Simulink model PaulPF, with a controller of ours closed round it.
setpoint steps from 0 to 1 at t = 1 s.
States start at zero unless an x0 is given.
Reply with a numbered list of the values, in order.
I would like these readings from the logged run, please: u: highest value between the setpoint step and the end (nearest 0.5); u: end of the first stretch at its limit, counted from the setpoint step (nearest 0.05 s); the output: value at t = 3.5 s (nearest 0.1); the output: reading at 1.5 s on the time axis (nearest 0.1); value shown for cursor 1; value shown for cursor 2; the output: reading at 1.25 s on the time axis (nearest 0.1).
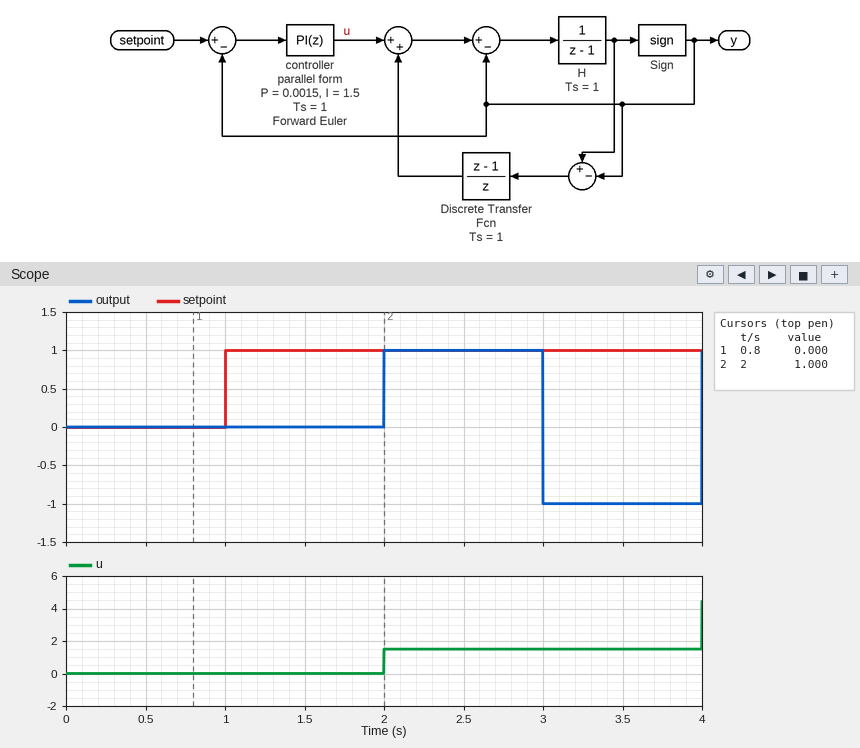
1. 1.5
2. 1.00 s
3. -1.0
4. 0.0
5. 0.000
6. 1.000
7. 0.0
